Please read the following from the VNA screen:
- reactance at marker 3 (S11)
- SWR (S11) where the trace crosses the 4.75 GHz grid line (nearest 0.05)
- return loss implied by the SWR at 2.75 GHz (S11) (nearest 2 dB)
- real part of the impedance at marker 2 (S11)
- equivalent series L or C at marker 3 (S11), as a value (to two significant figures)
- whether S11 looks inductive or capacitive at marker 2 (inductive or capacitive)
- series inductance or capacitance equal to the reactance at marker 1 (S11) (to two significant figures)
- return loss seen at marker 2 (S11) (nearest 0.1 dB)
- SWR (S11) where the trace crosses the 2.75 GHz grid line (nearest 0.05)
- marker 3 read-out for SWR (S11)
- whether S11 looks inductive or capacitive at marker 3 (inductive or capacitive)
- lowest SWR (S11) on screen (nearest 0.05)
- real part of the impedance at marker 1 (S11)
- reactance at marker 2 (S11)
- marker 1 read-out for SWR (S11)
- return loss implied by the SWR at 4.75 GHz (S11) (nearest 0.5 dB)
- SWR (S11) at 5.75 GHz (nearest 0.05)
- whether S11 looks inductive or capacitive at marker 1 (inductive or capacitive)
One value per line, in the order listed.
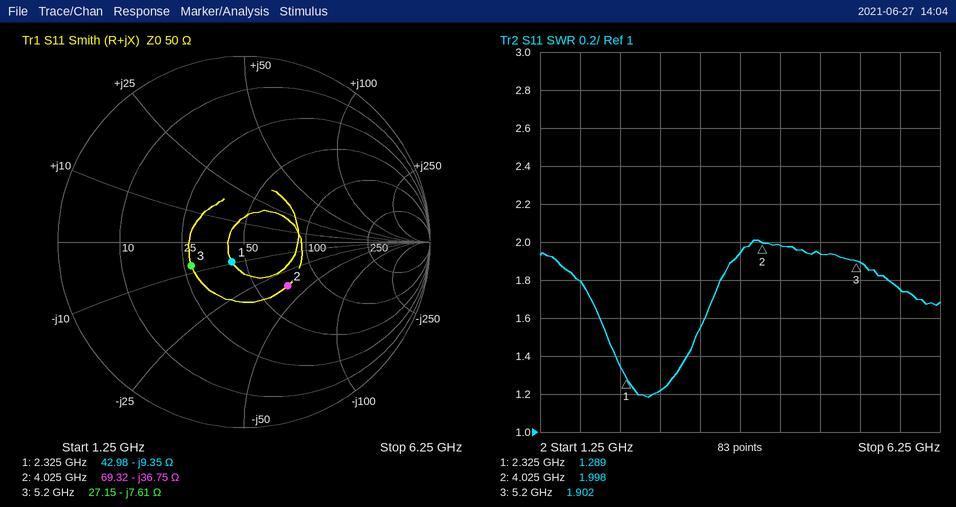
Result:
-7.61 Ω
1.95
20 dB
69.32 Ω
4.0 pF
capacitive
7.3 pF
9.6 dB
1.20
1.902
capacitive
1.20
42.98 Ω
-36.75 Ω
1.289
10.0 dB
1.75
capacitive
